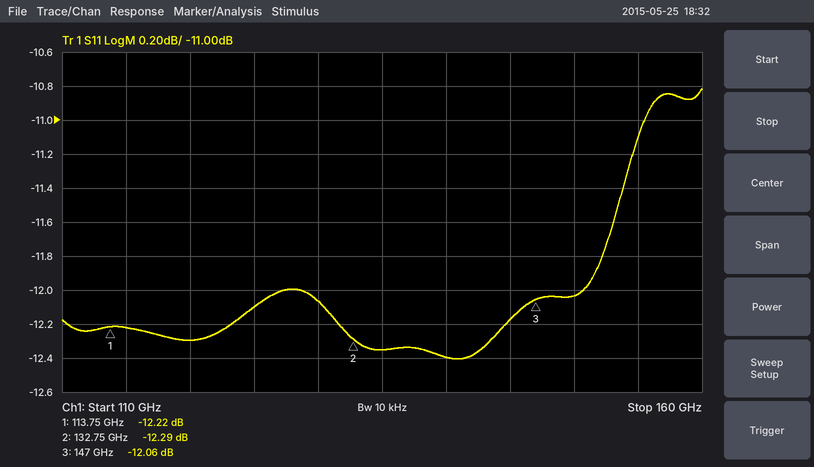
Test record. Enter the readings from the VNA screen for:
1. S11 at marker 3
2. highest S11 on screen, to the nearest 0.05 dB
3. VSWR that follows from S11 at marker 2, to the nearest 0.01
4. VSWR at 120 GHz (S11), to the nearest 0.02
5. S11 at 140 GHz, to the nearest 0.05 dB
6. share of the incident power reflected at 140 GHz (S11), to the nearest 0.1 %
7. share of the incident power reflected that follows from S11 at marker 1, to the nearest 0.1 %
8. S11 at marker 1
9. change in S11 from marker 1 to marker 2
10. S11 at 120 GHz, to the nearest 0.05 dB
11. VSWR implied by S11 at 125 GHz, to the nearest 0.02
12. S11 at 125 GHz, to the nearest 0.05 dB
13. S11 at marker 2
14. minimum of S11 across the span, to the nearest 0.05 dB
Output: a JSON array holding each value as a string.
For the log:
["-12.06 dB", "-10.80 dB", "1.64", "1.64", "-12.40 dB", "5.8 %", "6.0 %", "-12.22 dB", "-0.07 dB", "-12.30 dB", "1.66", "-12.10 dB", "-12.29 dB", "-12.40 dB"]
